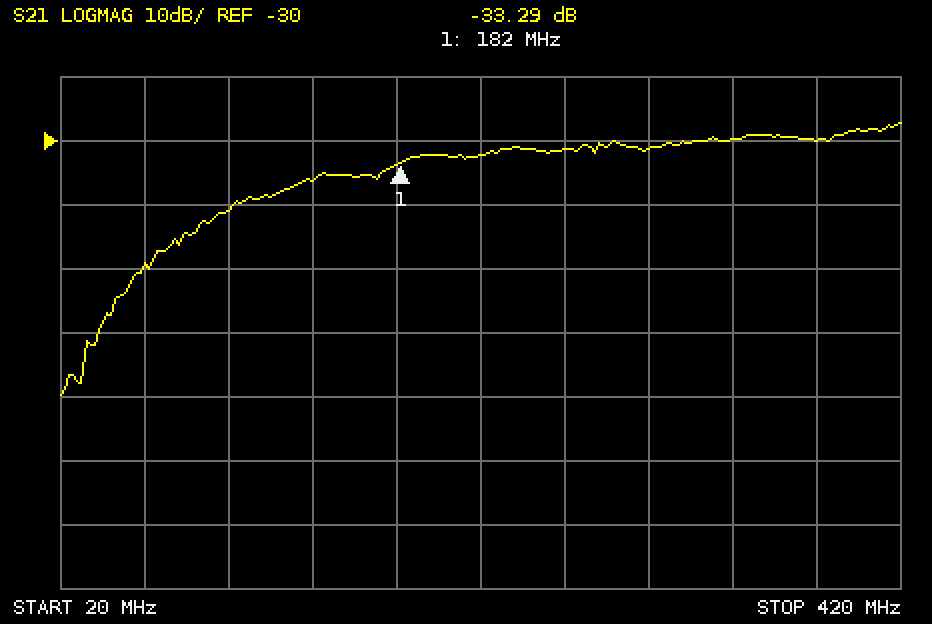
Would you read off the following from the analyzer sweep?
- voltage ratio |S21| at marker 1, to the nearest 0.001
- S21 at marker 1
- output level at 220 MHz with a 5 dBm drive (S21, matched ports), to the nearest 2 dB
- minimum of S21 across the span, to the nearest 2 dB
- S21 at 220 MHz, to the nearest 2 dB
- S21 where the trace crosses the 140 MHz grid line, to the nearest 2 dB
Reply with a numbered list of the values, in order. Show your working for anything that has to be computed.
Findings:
1. 10^(-33.29/20) ≈ 0.022
2. -33.29 dB
3. 5 dBm + (-32 dB) = -28 dBm
4. -70 dB
5. -32 dB
6. -36 dB
